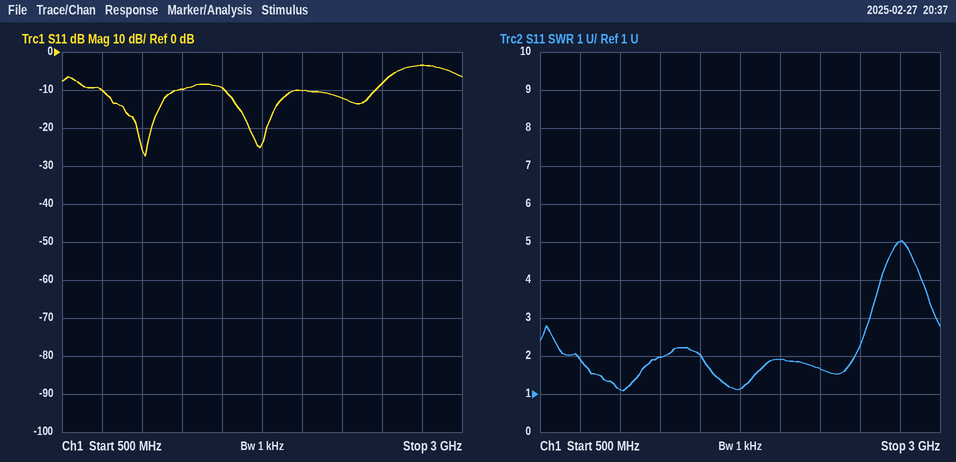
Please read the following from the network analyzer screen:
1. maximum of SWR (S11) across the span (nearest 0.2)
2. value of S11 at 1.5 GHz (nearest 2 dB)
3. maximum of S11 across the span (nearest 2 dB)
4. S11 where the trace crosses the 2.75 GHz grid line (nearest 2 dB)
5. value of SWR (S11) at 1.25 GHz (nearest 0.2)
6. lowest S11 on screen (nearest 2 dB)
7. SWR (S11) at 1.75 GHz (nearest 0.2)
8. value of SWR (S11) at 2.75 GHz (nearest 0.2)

5.0
-10 dB
-4 dB
-4 dB
2.0
-28 dB
1.2
5.0
